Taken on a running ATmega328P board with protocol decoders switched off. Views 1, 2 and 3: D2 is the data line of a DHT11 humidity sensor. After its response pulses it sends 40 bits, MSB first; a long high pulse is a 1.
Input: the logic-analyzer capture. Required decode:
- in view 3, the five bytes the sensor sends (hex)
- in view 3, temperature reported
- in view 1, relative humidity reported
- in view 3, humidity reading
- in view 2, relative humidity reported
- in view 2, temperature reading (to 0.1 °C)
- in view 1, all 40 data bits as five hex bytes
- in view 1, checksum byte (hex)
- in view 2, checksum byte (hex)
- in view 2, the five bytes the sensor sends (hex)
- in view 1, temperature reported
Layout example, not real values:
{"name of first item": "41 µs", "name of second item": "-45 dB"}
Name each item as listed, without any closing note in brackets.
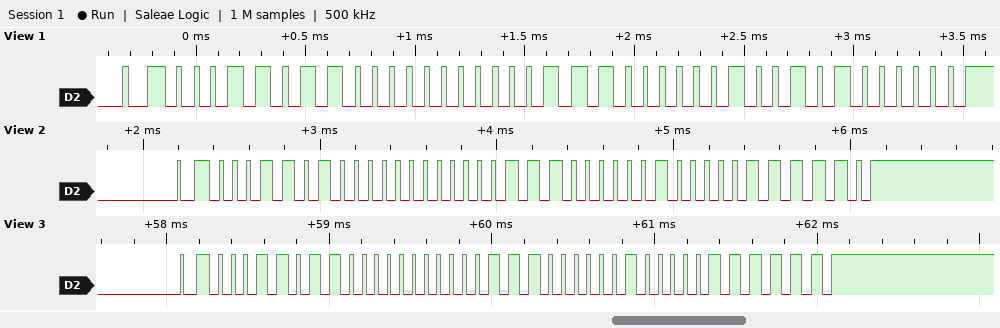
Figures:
{"in view 3, the five bytes the sensor sends": "1B 00 1C 08 3F", "in view 3, temperature reported": "28.8 °C", "in view 1, relative humidity reported": "27 %", "in view 3, humidity reading": "27 %", "in view 2, relative humidity reported": "26 %", "in view 2, temperature reading": "28.8 °C", "in view 1, all 40 data bits as five hex bytes": "1B 00 1C 09 40", "in view 1, checksum byte": "0x40", "in view 2, checksum byte": "0x3E", "in view 2, the five bytes the sensor sends": "1A 00 1C 08 3E", "in view 1, temperature reported": "28.9 °C"}
